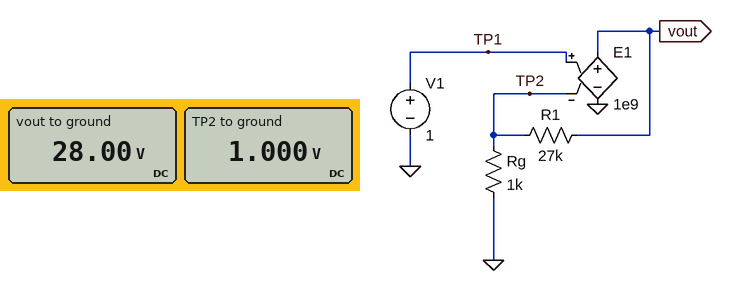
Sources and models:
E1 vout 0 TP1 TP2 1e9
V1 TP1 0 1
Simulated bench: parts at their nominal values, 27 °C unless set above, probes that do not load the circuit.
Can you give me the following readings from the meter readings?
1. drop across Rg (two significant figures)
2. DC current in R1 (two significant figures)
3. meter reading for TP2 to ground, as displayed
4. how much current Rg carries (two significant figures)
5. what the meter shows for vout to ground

1.0 V
1.0 mA
1.000 V
1.0 mA
28.00 V
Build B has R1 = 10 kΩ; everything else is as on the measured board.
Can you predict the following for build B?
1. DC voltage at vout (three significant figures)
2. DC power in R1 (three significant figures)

11.0 V
10.0 mW
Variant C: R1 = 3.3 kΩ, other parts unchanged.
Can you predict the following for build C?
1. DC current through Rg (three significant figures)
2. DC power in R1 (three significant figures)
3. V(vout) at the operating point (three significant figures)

1.00 mA
3.30 mW
4.30 V
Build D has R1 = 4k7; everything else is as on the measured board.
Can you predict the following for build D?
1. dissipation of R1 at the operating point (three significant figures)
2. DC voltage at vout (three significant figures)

4.70 mW
5.70 V
